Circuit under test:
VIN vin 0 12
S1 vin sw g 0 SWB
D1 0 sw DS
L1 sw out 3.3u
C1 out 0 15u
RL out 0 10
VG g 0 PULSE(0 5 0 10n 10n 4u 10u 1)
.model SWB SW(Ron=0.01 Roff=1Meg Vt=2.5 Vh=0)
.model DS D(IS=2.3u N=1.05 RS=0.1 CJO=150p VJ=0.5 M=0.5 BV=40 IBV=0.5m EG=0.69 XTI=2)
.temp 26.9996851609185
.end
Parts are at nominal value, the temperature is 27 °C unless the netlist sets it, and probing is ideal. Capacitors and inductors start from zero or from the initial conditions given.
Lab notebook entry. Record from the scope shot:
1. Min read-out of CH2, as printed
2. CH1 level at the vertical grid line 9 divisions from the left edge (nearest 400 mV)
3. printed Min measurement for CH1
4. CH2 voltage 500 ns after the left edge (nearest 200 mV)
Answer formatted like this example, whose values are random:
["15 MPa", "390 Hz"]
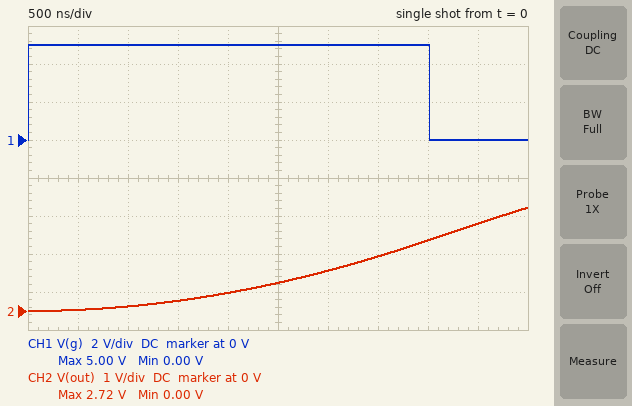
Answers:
["0.00 V", "0 V", "0.00 V", "0 V"]
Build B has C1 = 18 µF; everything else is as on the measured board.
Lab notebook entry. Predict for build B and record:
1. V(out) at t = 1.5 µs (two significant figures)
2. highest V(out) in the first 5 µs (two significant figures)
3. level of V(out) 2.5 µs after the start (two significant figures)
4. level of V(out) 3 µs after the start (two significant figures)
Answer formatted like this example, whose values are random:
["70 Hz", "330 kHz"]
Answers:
["220 mV", "2.3 V", "620 mV", "890 mV"]
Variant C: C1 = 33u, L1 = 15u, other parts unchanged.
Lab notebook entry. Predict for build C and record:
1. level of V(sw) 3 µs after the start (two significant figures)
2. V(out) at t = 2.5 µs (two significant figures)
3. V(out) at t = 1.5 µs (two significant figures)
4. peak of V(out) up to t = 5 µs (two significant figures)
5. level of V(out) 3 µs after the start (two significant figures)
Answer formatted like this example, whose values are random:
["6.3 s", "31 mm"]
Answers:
["12 V", "75 mV", "27 mV", "290 mV", "110 mV"]
